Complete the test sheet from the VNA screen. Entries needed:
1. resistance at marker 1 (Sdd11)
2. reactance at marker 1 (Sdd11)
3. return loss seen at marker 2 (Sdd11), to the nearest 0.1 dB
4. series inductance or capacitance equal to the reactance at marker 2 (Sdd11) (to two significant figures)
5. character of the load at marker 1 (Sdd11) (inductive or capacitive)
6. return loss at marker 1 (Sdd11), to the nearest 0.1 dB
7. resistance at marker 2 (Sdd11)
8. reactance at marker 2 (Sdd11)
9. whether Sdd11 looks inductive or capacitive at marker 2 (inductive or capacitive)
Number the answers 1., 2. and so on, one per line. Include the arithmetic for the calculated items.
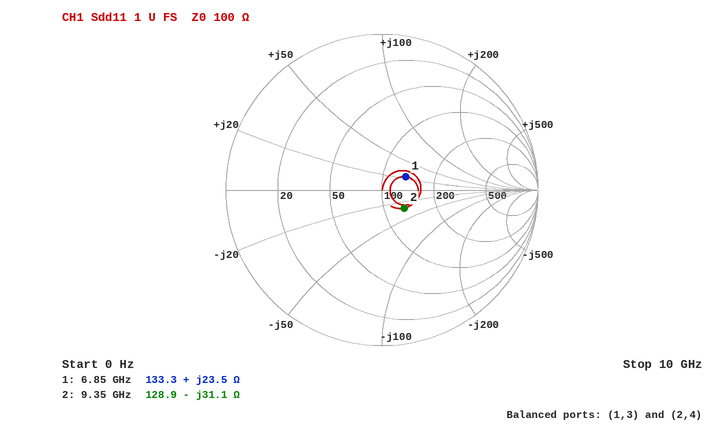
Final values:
1. 133.3 Ω
2. +23.5 Ω
3. 14.7 dB
4. C = 1/(2π × 9.35 GHz × 31.1 Ω) ≈ 547 fF, so 550 fF to two significant figures
5. inductive
6. 15.2 dB
7. 128.9 Ω
8. -31.1 Ω
9. capacitive
